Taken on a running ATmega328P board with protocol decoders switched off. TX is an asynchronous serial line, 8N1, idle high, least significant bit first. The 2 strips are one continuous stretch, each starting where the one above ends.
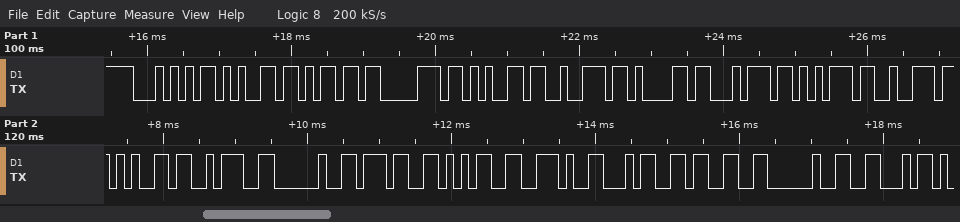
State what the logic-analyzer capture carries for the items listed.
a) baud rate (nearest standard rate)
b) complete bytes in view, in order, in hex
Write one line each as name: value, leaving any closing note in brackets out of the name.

baud rate: 9600 baud
complete bytes in view, in order, in hex: 54 65 6D 70 65 72 61 74 75 72 65 3A 20 37 35 2E 34 33 20 46
